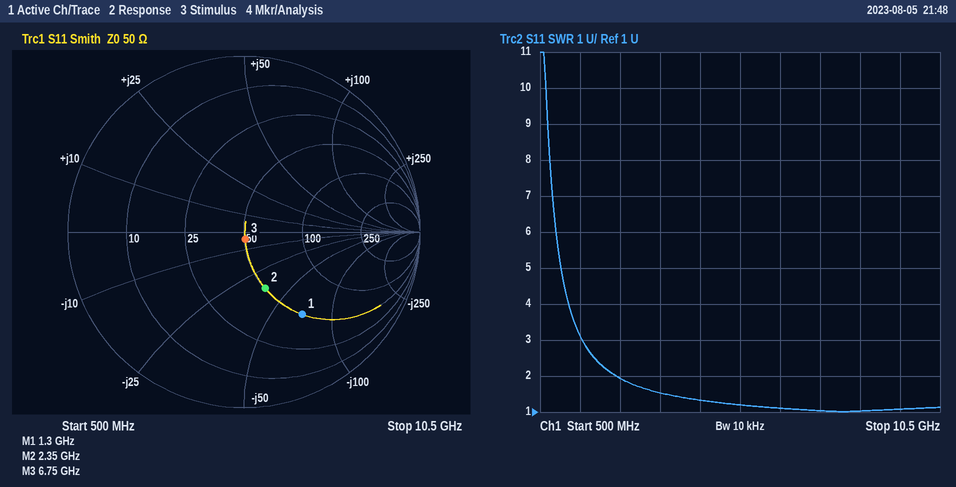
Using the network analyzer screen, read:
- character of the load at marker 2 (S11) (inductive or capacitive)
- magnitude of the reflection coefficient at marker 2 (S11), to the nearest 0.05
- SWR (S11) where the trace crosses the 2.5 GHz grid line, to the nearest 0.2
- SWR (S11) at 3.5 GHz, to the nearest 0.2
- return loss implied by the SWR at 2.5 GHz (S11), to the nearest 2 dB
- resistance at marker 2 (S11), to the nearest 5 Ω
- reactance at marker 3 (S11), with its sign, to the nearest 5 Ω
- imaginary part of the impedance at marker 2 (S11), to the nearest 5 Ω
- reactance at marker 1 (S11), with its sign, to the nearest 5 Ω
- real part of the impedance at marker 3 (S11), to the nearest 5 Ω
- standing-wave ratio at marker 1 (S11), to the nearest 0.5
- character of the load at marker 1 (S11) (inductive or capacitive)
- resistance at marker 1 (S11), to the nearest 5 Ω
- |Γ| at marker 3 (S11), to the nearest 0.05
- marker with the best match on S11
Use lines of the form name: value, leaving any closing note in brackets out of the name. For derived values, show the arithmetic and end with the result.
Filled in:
character of the load at marker 2 (S11): capacitive
magnitude of the reflection coefficient at marker 2 (S11), to the nearest 0.05: 0.35
SWR (S11) where the trace crosses the 2.5 GHz grid line, to the nearest 0.2: 2.0
SWR (S11) at 3.5 GHz, to the nearest 0.2: 1.6
return loss implied by the SWR at 2.5 GHz (S11), to the nearest 2 dB: −20 log10((2 − 1)/(2 + 1)) ≈ 10 dB
resistance at marker 2 (S11), to the nearest 5 Ω: 50 Ω
reactance at marker 3 (S11), with its sign, to the nearest 5 Ω: -5 Ω
imaginary part of the impedance at marker 2 (S11), to the nearest 5 Ω: -35 Ω
reactance at marker 1 (S11), with its sign, to the nearest 5 Ω: -70 Ω
real part of the impedance at marker 3 (S11), to the nearest 5 Ω: 50 Ω
standing-wave ratio at marker 1 (S11), to the nearest 0.5: 3.5
character of the load at marker 1 (S11): capacitive
resistance at marker 1 (S11), to the nearest 5 Ω: 50 Ω
|Γ| at marker 3 (S11), to the nearest 0.05: 0.05
marker with the best match on S11: marker 3
